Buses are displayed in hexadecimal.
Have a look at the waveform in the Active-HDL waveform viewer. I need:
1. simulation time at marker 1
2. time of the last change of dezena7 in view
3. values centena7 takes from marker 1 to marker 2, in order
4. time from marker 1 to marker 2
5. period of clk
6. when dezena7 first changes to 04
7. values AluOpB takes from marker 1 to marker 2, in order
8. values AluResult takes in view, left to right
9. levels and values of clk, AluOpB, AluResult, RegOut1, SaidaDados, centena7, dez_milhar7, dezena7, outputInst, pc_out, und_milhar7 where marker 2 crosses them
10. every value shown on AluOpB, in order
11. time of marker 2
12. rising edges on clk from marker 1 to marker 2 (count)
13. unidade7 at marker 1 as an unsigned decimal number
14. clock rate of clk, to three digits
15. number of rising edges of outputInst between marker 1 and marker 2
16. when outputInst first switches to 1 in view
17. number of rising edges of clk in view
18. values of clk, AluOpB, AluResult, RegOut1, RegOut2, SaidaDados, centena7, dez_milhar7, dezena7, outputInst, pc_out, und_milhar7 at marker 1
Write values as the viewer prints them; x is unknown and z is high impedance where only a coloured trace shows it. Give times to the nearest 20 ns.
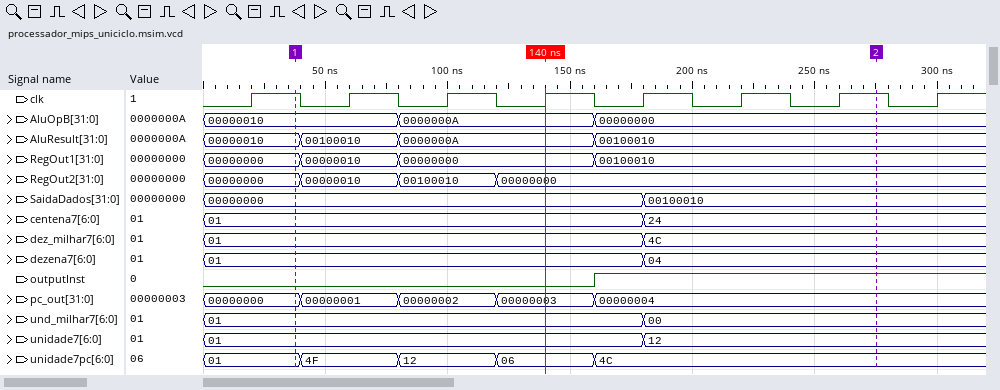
40 ns
180 ns
01, 24
240 ns
40 ns
180 ns
00000010, 0000000A, 00000000
00000010, 00100010, 0000000A, 00100010
clk=1, AluOpB=00000000, AluResult=00100010, RegOut1=00100010, SaidaDados=00100010, centena7=24, dez_milhar7=4C, dezena7=04, outputInst=1, pc_out=00000004, und_milhar7=00
00000010, 0000000A, 00000000
280 ns
6
1
25.0 MHz
1
160 ns
8
clk=1, AluOpB=00000010, AluResult=00000010, RegOut1=00000000, RegOut2=00000000, SaidaDados=00000000, centena7=01, dez_milhar7=01, dezena7=01, outputInst=0, pc_out=00000000, und_milhar7=01
